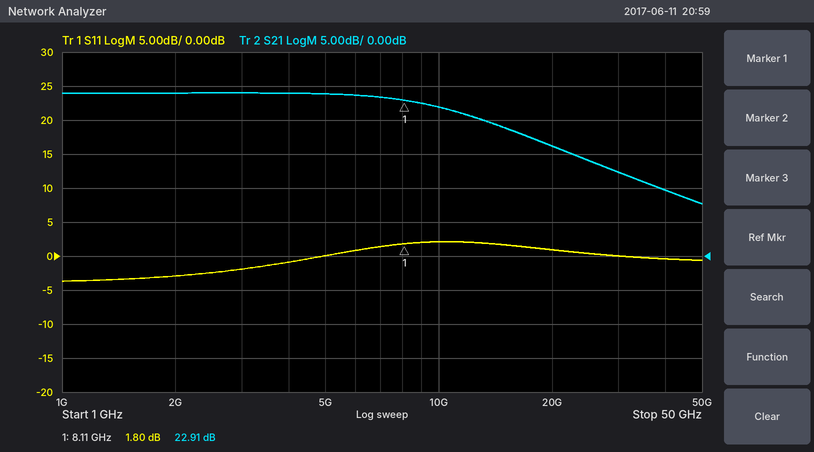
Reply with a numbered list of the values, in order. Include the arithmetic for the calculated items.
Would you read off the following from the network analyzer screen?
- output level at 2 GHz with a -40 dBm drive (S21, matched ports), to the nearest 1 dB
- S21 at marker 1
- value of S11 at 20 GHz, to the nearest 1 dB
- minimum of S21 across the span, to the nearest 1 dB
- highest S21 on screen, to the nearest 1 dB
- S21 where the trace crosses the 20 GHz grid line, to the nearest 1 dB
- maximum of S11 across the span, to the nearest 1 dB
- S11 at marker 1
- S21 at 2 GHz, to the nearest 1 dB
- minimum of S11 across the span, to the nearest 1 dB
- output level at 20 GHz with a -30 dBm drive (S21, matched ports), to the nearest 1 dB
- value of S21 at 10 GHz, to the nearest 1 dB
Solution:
1. -40 dBm + (24 dB) = -16 dBm
2. 22.91 dB
3. 1 dB
4. 8 dB
5. 24 dB
6. 16 dB
7. 2 dB
8. 1.80 dB
9. 24 dB
10. -4 dB
11. -30 dBm + (16 dB) = -14 dBm
12. 22 dB
